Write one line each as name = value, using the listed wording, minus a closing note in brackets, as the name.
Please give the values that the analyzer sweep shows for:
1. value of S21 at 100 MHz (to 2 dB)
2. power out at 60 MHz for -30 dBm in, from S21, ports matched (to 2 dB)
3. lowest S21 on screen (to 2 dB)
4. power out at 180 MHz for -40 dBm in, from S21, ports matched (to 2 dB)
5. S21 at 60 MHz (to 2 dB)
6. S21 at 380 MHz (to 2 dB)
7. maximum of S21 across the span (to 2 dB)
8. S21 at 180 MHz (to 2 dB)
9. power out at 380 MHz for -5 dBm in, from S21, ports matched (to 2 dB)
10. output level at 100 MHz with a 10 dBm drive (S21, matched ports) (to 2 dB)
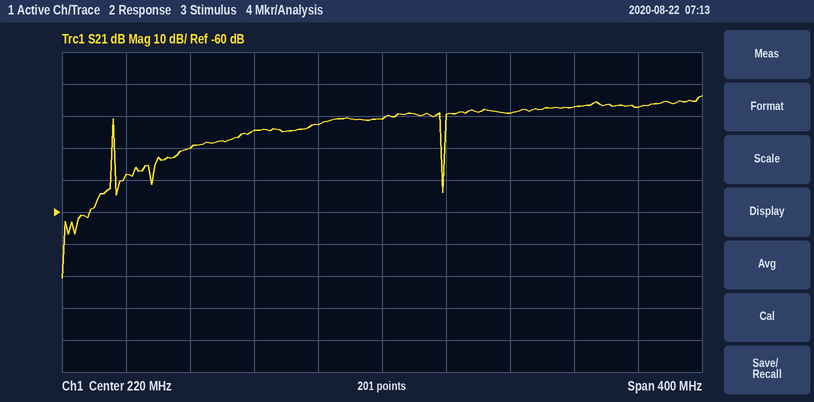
value of S21 at 100 MHz = -40 dB
power out at 60 MHz for -30 dBm in, from S21, ports matched = -78 dBm
lowest S21 on screen = -80 dB
power out at 180 MHz for -40 dBm in, from S21, ports matched = -72 dBm
S21 at 60 MHz = -48 dB
S21 at 380 MHz = -28 dB
maximum of S21 across the span = -24 dB
S21 at 180 MHz = -32 dB
power out at 380 MHz for -5 dBm in, from S21, ports matched = -32 dBm
output level at 100 MHz with a 10 dBm drive (S21, matched ports) = -30 dBm
